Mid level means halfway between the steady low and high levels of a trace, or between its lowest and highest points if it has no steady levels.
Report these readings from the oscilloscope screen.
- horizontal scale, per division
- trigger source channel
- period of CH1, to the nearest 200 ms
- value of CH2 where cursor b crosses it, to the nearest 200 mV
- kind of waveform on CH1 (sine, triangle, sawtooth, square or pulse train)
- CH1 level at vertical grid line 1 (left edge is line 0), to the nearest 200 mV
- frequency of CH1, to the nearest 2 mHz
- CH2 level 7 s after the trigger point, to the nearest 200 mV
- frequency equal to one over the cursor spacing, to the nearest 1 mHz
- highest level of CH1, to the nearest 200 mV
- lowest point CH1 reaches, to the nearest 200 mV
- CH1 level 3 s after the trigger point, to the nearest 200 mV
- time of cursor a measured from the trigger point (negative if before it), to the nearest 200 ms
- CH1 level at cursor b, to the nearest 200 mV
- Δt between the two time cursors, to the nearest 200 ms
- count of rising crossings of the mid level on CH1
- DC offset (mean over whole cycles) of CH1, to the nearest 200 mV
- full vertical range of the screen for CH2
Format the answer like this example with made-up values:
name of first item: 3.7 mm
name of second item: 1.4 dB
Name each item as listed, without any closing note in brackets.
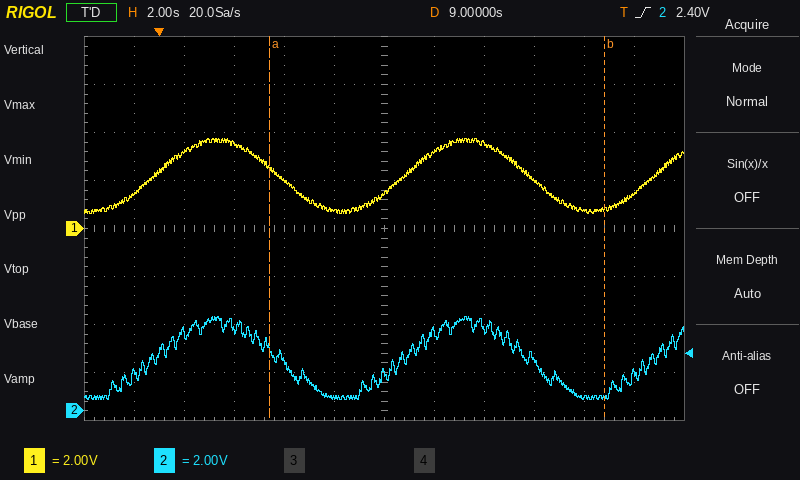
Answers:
horizontal scale, per division: 2 s
trigger source channel: CH2
period of CH1, to the nearest 200 ms: 10.0 s
value of CH2 where cursor b crosses it, to the nearest 200 mV: 600 mV
kind of waveform on CH1: sine
CH1 level at vertical grid line 1 (left edge is line 0), to the nearest 200 mV: 1.4 V
frequency of CH1, to the nearest 2 mHz: 100 mHz
CH2 level 7 s after the trigger point, to the nearest 200 mV: 600 mV
frequency equal to one over the cursor spacing, to the nearest 1 mHz: 75 mHz
highest level of CH1, to the nearest 200 mV: 3.8 V
lowest point CH1 reaches, to the nearest 200 mV: 600 mV
CH1 level 3 s after the trigger point, to the nearest 200 mV: 3.6 V
time of cursor a measured from the trigger point (negative if before it), to the nearest 200 ms: +4.4 s
CH1 level at cursor b, to the nearest 200 mV: 800 mV
Δt between the two time cursors, to the nearest 200 ms: 13.4 s
count of rising crossings of the mid level on CH1: 3
DC offset (mean over whole cycles) of CH1, to the nearest 200 mV: 2.2 V
full vertical range of the screen for CH2: 16 V
